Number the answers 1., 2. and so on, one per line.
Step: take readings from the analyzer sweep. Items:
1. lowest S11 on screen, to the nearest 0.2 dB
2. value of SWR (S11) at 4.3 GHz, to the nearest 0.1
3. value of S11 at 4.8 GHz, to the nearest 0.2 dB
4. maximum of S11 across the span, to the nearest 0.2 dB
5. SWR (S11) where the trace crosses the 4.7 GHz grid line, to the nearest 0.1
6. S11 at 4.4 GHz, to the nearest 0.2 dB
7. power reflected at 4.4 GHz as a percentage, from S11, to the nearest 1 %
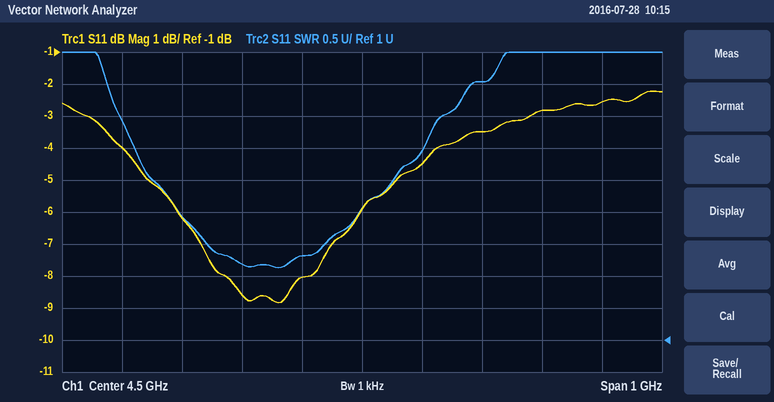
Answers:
1. -8.8 dB
2. 2.2
3. -2.8 dB
4. -2.2 dB
5. 5.0
6. -8.0 dB
7. 16 %
